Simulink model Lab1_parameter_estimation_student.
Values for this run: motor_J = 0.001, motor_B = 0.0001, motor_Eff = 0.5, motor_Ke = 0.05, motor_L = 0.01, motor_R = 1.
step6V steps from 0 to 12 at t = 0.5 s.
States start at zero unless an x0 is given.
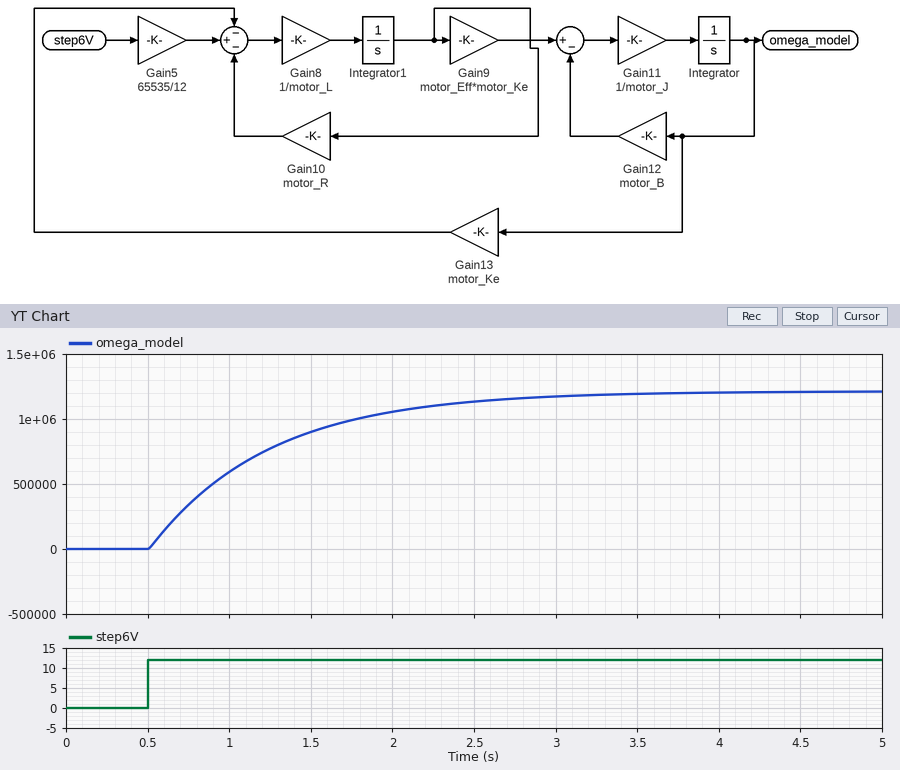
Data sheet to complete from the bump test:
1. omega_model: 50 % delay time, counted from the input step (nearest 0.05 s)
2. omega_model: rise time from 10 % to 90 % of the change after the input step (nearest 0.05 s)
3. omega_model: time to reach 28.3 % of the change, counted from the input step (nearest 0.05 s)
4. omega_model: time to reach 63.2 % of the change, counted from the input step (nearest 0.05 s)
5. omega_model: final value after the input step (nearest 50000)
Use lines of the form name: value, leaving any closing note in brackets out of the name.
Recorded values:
omega_model: 50 % delay time, counted from the input step: 0.50 s
omega_model: rise time from 10 % to 90 % of the change after the input step: 1.60 s
omega_model: time to reach 28.3 % of the change, counted from the input step: 0.25 s
omega_model: time to reach 63.2 % of the change, counted from the input step: 0.75 s
omega_model: final value after the input step: 1200000
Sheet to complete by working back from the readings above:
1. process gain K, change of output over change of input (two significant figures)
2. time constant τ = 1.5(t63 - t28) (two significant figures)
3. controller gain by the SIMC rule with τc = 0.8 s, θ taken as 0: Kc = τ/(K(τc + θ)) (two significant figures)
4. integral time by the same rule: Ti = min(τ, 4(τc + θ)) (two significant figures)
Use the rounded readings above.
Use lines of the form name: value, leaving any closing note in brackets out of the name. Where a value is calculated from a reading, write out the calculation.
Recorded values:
process gain K, change of output over change of input: (1.2e+06 - 0) / 12 = 100000
time constant τ = 1.5(t63 - t28): 1.5 × (0.75 - 0.25) = 0.75 s
controller gain by the SIMC rule with τc = 0.8 s, θ taken as 0: Kc = τ/(K(τc + θ)): 0.75 / (100000 × (0.8 + 0)) = 0.0000094
integral time by the same rule: Ti = min(τ, 4(τc + θ)): min(0.75, 4 × (0.8 + 0)) = 0.75 s
